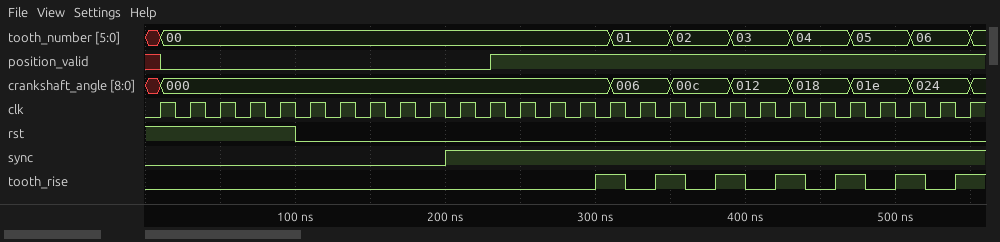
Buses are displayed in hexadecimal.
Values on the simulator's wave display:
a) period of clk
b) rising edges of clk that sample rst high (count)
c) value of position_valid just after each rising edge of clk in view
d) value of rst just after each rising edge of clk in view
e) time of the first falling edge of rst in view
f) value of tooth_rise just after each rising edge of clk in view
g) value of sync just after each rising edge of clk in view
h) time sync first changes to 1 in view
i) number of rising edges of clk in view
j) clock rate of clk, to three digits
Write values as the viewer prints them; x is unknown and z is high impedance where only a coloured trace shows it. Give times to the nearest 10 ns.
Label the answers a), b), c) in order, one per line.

a) 20 ns
b) 5
c) 0 0 0 0 0 0 0 0 0 0 0 1 1 1 1 1 1 1 1 1 1 1 1 1 1 1 1 1
d) 1 1 1 1 1 0 0 0 0 0 0 0 0 0 0 0 0 0 0 0 0 0 0 0 0 0 0 0
e) 100 ns
f) 0 0 0 0 0 0 0 0 0 0 0 0 0 0 0 1 0 1 0 1 0 1 0 1 0 1 0 1
g) 0 0 0 0 0 0 0 0 0 0 1 1 1 1 1 1 1 1 1 1 1 1 1 1 1 1 1 1
h) 200 ns
i) 28
j) 50.0 MHz
